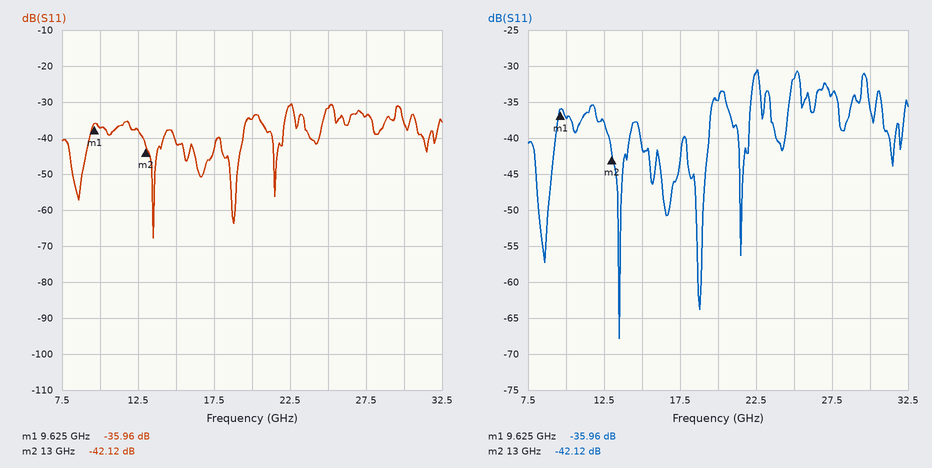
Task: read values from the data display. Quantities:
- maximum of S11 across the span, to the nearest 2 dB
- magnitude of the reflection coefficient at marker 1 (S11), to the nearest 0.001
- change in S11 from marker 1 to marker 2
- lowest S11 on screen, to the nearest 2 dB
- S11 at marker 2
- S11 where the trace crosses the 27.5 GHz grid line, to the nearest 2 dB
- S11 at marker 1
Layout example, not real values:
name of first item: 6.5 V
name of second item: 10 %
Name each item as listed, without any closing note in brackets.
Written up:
maximum of S11 across the span, to the nearest 2 dB: -30 dB
magnitude of the reflection coefficient at marker 1 (S11), to the nearest 0.001: 0.016
change in S11 from marker 1 to marker 2: -6.16 dB
lowest S11 on screen, to the nearest 2 dB: -68 dB
S11 at marker 2: -42.12 dB
S11 where the trace crosses the 27.5 GHz grid line, to the nearest 2 dB: -34 dB
S11 at marker 1: -35.96 dB
